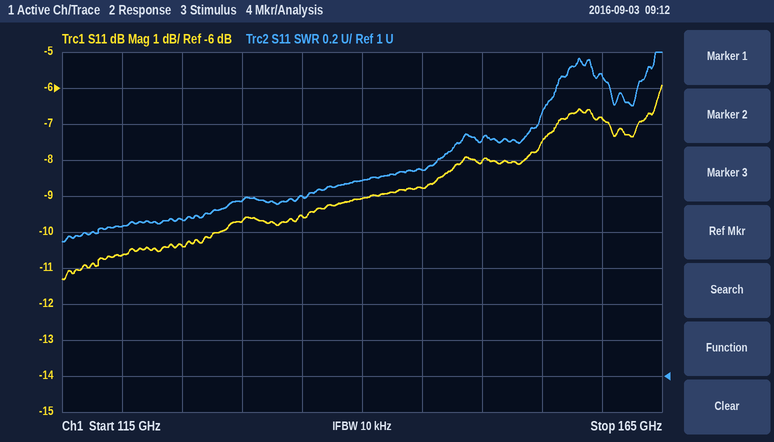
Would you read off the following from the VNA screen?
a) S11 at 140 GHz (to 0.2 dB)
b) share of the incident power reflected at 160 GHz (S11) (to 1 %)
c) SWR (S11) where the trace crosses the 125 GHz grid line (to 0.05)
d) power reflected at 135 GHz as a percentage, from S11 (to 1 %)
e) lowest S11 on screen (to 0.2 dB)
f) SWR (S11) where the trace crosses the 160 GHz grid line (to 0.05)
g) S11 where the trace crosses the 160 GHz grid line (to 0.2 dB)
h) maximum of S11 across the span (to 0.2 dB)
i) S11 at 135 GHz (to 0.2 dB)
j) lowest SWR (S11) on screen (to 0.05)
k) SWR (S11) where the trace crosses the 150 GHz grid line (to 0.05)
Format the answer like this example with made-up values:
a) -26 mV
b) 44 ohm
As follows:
a) -9.0 dB
b) 21 %
c) 1.85
d) 11 %
e) -11.4 dB
f) 2.65
g) -6.8 dB
h) -6.0 dB
i) -9.6 dB
j) 1.75
k) 2.30
